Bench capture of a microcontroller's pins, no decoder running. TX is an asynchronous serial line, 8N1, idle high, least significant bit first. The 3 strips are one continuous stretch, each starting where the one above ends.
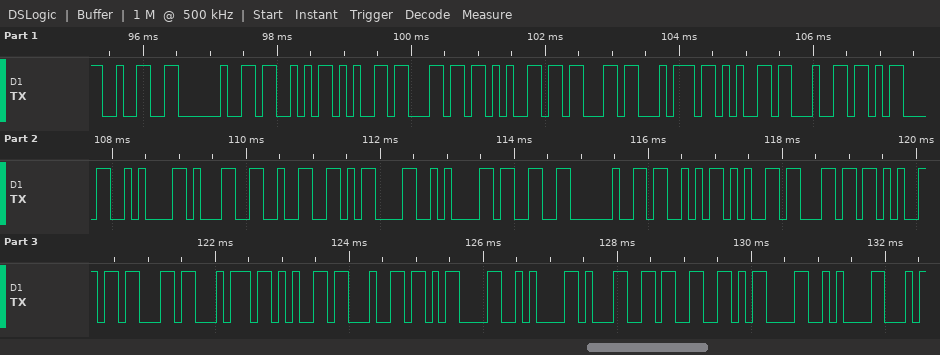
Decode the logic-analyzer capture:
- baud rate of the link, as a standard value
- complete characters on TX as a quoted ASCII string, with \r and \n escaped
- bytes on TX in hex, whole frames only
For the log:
9600 baud
"2 Selected\r\n12\r\n3 Selected\r\n13\r\n"
32 20 53 65 6C 65 63 74 65 64 0D 0A 31 32 0D 0A 33 20 53 65 6C 65 63 74 65 64 0D 0A 31 33 0D 0A
